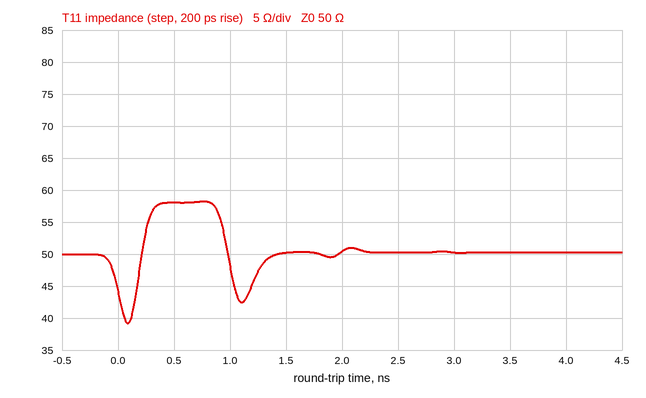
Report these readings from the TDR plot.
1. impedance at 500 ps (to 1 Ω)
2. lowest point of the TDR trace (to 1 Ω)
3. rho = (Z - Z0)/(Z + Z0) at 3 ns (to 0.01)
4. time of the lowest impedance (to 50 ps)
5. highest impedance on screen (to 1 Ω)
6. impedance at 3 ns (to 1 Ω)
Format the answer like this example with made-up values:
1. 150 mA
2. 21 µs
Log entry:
1. 58 Ω
2. 39 Ω
3. 0.00
4. 100 ps
5. 58 Ω
6. 50 Ω
